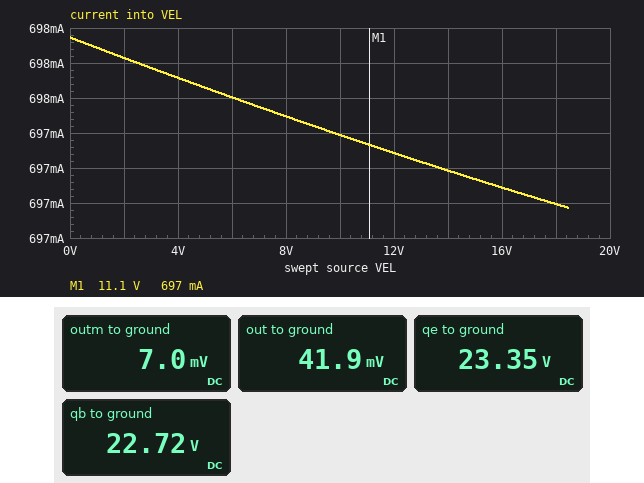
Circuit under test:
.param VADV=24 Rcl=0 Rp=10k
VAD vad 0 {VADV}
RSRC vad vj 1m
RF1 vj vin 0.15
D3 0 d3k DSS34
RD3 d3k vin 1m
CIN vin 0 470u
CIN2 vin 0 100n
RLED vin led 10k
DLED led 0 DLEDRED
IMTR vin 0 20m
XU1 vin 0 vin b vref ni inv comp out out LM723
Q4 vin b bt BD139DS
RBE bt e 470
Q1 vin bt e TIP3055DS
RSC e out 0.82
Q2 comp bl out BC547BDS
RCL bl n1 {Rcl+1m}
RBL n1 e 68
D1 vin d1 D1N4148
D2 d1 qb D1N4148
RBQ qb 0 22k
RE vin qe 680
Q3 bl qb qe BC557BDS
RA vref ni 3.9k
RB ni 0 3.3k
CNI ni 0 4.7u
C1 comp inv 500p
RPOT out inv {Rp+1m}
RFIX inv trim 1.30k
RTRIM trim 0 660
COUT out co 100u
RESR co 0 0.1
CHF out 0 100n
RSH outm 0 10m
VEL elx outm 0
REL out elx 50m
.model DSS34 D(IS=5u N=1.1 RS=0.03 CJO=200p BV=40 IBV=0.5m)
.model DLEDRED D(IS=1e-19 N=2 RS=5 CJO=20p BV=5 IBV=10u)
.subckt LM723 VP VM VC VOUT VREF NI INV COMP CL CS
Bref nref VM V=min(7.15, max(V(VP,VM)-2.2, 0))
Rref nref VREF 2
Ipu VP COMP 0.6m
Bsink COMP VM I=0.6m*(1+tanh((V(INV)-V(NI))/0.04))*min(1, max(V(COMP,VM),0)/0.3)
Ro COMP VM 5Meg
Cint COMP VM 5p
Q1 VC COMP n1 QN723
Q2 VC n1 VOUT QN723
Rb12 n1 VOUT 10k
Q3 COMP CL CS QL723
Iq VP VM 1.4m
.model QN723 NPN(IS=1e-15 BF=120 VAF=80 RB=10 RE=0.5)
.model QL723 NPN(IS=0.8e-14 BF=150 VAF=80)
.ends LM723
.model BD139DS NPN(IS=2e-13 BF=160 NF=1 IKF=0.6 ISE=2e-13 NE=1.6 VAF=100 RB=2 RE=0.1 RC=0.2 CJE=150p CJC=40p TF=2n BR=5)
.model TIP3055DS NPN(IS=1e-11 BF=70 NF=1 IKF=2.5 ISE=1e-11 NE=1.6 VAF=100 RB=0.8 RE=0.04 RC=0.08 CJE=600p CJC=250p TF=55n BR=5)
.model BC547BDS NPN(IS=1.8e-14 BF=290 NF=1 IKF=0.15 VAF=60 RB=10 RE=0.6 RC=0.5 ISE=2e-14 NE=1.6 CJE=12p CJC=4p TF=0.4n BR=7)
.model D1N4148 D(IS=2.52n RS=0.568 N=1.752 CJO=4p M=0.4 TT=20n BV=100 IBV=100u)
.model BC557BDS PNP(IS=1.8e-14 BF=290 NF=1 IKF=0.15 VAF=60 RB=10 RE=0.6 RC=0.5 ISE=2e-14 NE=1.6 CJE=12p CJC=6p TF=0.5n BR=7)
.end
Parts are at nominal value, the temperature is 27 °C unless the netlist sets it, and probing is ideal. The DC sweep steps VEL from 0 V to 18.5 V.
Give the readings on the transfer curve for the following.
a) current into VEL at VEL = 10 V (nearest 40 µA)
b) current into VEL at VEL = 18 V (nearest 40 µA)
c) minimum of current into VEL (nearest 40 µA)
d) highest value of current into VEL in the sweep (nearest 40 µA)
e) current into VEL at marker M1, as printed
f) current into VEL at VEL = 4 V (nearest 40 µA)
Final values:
697.40 mA
697.00 mA
696.96 mA
697.96 mA
697 mA
697.72 mA
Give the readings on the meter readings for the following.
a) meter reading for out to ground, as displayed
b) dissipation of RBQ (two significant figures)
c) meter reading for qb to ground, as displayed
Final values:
41.9 mV
23 mW
22.72 V
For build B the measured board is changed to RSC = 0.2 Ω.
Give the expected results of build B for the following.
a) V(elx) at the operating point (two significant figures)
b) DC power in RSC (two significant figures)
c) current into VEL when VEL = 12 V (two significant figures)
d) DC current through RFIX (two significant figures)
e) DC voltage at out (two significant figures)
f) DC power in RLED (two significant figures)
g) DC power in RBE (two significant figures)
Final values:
29 mV
1.6 W
2.9 A
14 µA
170 mV
47 mW
1.6 mW
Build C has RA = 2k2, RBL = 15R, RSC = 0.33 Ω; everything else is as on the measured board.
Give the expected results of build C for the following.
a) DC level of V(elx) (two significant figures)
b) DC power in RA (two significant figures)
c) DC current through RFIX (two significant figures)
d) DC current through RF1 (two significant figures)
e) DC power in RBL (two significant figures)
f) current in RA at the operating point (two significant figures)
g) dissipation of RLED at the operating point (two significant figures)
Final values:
19 mV
3.7 mW
9.3 µA
1.9 A
9.5 µW
1.3 mA
47 mW
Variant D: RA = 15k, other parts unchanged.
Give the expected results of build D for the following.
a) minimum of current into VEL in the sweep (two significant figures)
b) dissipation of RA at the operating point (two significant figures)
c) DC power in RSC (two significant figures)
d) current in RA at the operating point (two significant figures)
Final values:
-1.4 mA
2.3 mW
400 mW
390 µA
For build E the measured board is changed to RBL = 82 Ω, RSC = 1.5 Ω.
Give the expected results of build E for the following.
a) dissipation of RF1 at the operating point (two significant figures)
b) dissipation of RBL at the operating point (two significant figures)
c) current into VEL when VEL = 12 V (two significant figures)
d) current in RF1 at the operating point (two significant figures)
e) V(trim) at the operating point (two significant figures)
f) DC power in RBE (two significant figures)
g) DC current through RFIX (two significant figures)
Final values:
24 mW
52 µW
370 mA
400 mA
1.2 mV
890 µW
1.9 µA
